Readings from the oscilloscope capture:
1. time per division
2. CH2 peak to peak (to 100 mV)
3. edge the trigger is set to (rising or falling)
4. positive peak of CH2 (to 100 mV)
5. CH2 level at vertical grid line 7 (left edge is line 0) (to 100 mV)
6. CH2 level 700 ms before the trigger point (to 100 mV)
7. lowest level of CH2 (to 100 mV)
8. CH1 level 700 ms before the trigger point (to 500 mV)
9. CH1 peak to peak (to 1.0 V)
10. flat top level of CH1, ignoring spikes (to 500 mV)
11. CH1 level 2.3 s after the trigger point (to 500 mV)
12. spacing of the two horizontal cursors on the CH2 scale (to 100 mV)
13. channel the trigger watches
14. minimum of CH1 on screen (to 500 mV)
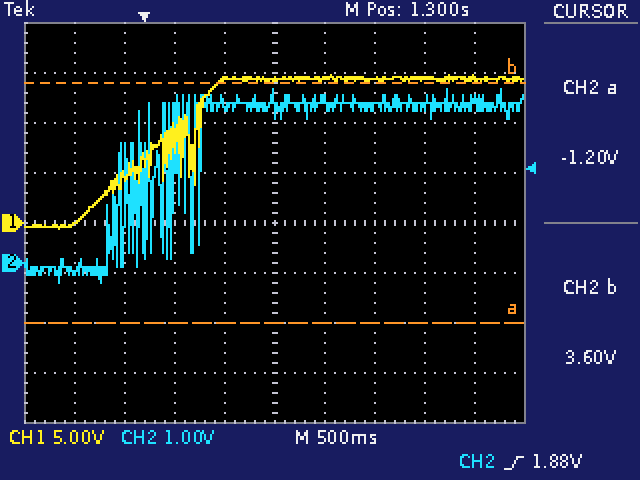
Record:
500 ms
3.9 V
rising
3.5 V
3.1 V
-200 mV
-400 mV
0.0 V
15.0 V
14.5 V
14.5 V
4.8 V
CH2
-500 mV
